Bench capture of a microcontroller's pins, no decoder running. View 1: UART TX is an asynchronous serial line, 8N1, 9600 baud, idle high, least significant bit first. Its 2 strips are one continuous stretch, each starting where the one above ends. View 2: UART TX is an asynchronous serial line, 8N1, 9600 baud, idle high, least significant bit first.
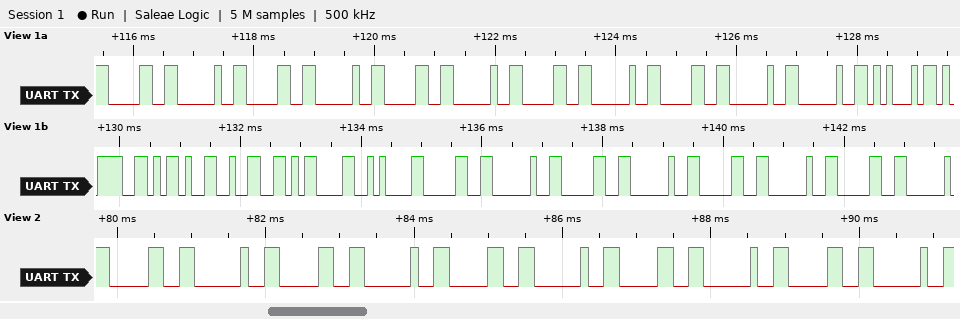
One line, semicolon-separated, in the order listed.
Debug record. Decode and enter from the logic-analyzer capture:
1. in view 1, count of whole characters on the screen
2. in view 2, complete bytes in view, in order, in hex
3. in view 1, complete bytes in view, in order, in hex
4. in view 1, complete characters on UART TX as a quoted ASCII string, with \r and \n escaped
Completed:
24; 30 20 30 20 30 20 30 20 30 20; 30 20 30 20 30 20 30 20 30 20 20 45 3D 2D 32 0D 0A 30 20 30 20 30 20 30; "0 0 0 0 0  E=-2\r\n0 0 0 0"
